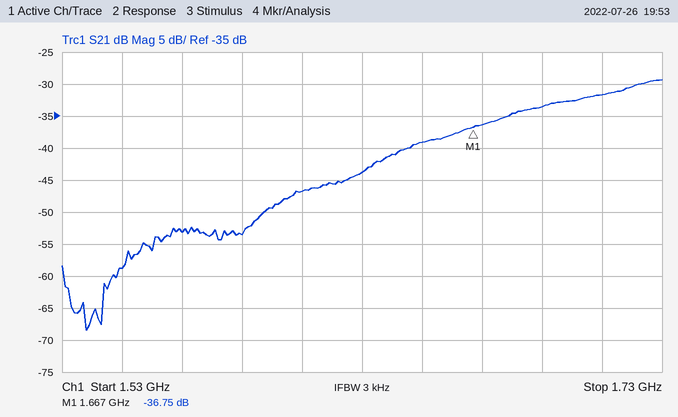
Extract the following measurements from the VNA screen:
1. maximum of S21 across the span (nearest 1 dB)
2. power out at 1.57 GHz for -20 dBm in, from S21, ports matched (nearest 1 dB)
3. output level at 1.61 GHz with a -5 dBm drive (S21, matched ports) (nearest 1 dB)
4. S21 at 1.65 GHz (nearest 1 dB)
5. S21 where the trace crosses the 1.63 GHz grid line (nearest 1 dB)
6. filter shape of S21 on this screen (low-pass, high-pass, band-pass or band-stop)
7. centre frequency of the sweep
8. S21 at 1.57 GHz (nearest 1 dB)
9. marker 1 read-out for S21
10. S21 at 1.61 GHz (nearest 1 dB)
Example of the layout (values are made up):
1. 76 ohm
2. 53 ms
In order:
1. -29 dB
2. -73 dBm
3. -52 dBm
4. -39 dB
5. -44 dB
6. high-pass
7. 1.63 GHz
8. -53 dB
9. -36.75 dB
10. -47 dB
